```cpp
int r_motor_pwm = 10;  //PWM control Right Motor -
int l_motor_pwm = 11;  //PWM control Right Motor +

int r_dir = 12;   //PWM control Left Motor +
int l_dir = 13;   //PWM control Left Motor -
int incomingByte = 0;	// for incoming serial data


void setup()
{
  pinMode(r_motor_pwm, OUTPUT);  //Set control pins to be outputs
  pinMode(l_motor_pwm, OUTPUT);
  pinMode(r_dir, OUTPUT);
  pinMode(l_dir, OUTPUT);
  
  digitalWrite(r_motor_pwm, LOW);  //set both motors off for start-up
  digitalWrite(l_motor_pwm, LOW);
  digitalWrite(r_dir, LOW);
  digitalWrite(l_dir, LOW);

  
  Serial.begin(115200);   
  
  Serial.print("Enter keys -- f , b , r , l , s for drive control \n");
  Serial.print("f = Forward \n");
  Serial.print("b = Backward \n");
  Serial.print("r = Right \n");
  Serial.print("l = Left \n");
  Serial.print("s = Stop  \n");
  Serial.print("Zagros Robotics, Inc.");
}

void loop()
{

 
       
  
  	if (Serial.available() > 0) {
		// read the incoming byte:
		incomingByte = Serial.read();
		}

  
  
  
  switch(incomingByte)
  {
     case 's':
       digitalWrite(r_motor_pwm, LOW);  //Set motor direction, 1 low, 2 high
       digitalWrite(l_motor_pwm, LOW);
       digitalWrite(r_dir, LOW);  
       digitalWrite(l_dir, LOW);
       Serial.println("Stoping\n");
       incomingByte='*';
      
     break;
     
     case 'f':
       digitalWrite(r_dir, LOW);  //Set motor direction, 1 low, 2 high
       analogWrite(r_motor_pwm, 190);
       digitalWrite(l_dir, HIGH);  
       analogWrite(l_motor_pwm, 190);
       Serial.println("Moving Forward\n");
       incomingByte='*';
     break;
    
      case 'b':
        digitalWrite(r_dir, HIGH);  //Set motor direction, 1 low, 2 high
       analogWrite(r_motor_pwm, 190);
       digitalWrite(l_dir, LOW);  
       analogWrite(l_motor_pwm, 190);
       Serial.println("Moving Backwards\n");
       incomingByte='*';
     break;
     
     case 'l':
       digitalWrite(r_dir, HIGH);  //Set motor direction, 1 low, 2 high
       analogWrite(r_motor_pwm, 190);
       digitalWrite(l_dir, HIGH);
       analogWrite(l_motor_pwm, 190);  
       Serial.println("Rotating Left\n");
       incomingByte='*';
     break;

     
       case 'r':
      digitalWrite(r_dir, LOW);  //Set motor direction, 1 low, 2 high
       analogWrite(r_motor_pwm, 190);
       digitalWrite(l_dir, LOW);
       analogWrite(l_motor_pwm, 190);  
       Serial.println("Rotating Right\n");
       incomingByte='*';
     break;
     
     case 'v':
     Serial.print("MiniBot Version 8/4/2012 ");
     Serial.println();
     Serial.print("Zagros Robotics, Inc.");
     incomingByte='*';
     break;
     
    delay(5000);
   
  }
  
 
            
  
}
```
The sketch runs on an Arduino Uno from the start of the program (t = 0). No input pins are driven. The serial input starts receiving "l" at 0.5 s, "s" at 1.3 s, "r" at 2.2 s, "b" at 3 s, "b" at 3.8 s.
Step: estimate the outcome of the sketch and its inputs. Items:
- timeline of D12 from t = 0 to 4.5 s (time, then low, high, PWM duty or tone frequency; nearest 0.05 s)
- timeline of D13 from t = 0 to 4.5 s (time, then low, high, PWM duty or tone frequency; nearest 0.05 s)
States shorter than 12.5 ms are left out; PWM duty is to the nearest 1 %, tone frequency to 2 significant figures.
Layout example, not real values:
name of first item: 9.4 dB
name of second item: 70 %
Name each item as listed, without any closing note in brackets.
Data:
timeline of D12 from t = 0 to 4.5 s: 0 s low; 0.5 s high; 1.3 s low; 3 s high
timeline of D13 from t = 0 to 4.5 s: 0 s low; 0.5 s high; 1.3 s low
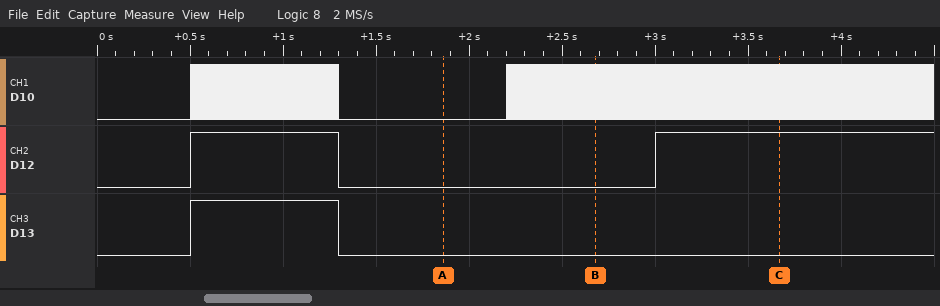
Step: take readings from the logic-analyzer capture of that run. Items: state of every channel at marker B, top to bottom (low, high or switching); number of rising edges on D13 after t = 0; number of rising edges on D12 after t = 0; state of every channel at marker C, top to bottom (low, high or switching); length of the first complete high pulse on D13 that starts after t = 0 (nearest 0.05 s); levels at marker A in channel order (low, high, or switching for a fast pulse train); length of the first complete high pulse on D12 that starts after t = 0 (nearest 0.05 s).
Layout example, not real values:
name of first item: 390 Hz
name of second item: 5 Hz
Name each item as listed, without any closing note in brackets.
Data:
state of every channel at marker B, top to bottom: D10 switching, D12 low, D13 low
number of rising edges on D13 after t = 0: 1
number of rising edges on D12 after t = 0: 2
state of every channel at marker C, top to bottom: D10 switching, D12 high, D13 low
length of the first complete high pulse on D13 that starts after t = 0: 0.80 s
levels at marker A in channel order: D10 low, D12 low, D13 low
length of the first complete high pulse on D12 that starts after t = 0: 0.80 s
